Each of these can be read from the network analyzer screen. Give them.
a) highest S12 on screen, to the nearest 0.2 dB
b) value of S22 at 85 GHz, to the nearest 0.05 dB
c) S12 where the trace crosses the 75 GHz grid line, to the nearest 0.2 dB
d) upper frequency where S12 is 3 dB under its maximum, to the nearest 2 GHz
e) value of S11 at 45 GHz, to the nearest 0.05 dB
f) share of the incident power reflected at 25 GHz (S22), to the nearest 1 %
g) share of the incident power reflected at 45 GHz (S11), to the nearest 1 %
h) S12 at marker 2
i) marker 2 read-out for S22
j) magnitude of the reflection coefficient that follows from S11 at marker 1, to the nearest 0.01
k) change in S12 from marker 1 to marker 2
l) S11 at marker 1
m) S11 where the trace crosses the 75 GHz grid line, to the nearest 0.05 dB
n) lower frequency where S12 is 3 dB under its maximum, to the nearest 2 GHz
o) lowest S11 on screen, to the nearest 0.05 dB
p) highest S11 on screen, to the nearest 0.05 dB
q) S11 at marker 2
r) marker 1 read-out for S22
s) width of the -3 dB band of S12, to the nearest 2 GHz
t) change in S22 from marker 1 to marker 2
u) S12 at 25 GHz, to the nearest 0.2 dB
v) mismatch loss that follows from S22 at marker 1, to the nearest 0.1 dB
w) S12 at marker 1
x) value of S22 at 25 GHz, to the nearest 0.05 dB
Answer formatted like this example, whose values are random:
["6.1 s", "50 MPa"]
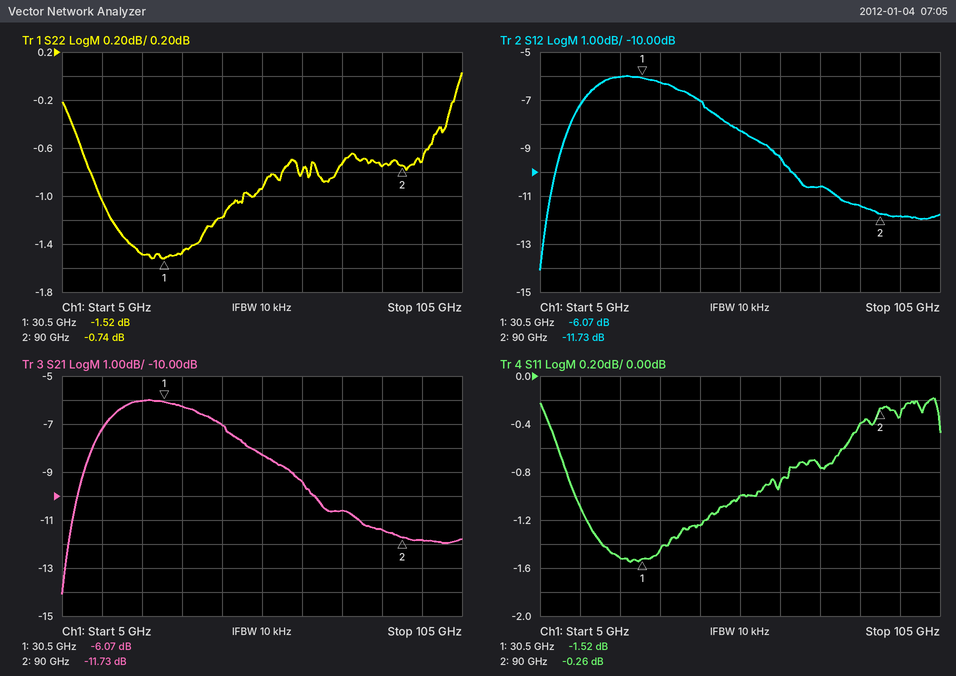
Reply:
["-6.0 dB", "-0.75 dB", "-10.6 dB", "62 GHz", "-1.25 dB", "71 %", "75 %", "-11.73 dB", "-0.74 dB", "0.84", "-5.66 dB", "-1.52 dB", "-0.75 dB", "10 GHz", "-1.55 dB", "-0.20 dB", "-0.26 dB", "-1.52 dB", "52 GHz", "0.78 dB", "-6.0 dB", "5.3 dB", "-6.07 dB", "-1.50 dB"]
